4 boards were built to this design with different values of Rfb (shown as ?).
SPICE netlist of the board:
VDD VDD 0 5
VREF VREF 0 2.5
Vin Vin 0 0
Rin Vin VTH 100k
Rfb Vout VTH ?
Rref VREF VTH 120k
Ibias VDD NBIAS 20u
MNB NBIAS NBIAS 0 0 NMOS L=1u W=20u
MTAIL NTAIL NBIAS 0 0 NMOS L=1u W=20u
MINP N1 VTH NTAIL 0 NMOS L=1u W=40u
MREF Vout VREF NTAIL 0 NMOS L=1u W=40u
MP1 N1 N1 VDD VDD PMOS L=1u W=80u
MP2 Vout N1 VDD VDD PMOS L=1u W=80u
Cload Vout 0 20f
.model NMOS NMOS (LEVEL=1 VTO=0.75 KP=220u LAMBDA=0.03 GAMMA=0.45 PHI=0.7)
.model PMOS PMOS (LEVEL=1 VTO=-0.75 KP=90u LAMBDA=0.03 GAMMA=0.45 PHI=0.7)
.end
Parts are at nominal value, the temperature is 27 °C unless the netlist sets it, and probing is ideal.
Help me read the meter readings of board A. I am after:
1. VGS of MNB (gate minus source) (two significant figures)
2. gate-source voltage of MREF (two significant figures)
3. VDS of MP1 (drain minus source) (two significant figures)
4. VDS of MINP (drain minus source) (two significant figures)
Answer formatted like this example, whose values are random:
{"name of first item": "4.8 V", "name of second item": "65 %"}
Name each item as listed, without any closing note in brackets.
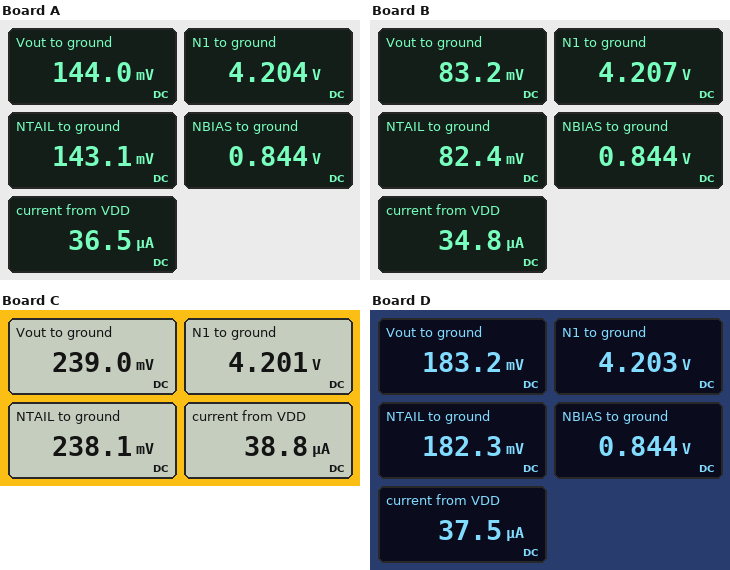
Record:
{"VGS of MNB (gate minus source)": "840 mV", "gate-source voltage of MREF": "2.4 V", "VDS of MP1 (drain minus source)": "-800 mV", "VDS of MINP (drain minus source)": "4.1 V"}
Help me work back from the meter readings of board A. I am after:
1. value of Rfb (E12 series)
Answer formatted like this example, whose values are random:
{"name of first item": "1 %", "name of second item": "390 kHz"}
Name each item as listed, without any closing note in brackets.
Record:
{"value of Rfb": "270 kΩ"}
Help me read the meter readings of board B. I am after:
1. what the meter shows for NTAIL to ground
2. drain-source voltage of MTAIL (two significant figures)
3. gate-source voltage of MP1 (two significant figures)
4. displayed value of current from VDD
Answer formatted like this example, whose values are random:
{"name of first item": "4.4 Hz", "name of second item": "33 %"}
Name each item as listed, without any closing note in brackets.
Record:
{"what the meter shows for NTAIL to ground": "82.4 mV", "drain-source voltage of MTAIL": "82 mV", "gate-source voltage of MP1": "-790 mV", "displayed value of current from VDD": "34.8 µA"}
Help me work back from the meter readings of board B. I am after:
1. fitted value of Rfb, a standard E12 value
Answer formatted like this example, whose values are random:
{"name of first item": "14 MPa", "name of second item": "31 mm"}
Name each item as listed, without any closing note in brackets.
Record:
{"fitted value of Rfb, a standard E12 value": "180 kΩ"}
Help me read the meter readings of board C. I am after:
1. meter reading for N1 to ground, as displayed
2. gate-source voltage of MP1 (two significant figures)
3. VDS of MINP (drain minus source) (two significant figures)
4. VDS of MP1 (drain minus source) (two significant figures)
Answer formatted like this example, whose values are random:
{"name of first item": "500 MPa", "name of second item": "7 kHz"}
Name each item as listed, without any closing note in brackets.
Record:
{"meter reading for N1 to ground, as displayed": "4.201 V", "gate-source voltage of MP1": "-800 mV", "VDS of MINP (drain minus source)": "4.0 V", "VDS of MP1 (drain minus source)": "-800 mV"}
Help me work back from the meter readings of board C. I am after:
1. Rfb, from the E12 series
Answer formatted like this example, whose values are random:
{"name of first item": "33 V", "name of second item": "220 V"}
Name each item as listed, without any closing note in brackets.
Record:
{"Rfb, from the E12 series": "1 MΩ"}
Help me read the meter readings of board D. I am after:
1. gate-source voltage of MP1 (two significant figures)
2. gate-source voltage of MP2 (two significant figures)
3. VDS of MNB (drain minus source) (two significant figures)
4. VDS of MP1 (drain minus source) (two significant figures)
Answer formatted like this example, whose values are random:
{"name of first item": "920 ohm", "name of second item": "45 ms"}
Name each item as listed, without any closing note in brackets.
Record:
{"gate-source voltage of MP1": "-800 mV", "gate-source voltage of MP2": "-800 mV", "VDS of MNB (drain minus source)": "840 mV", "VDS of MP1 (drain minus source)": "-800 mV"}
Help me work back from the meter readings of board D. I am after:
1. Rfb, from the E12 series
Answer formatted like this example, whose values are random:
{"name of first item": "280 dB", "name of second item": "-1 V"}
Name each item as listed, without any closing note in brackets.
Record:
{"Rfb, from the E12 series": "390 kΩ"}
